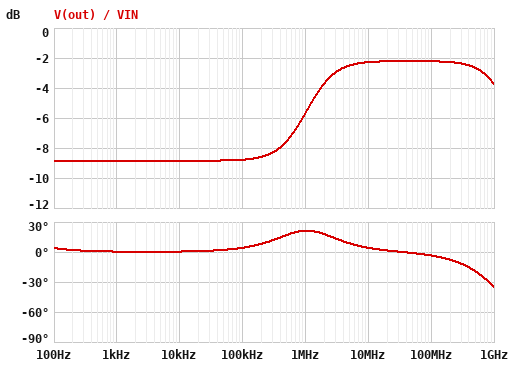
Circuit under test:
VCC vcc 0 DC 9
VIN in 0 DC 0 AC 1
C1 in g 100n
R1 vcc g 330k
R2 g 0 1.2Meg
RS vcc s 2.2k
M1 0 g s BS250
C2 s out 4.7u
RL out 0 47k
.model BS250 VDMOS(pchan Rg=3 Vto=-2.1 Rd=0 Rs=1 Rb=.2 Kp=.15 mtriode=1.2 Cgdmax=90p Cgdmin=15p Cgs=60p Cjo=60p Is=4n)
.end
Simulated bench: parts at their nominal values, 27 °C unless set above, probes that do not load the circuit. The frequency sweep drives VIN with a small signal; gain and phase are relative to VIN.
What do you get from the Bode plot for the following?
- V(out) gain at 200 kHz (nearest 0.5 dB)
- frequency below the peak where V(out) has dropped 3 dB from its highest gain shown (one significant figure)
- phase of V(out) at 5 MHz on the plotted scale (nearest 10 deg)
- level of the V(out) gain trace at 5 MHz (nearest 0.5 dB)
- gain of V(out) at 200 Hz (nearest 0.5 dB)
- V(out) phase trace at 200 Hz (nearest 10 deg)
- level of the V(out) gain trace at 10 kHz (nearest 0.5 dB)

-8.5 dB
1 MHz
10 deg
-2.5 dB
-9.0 dB
0 deg
-9.0 dB
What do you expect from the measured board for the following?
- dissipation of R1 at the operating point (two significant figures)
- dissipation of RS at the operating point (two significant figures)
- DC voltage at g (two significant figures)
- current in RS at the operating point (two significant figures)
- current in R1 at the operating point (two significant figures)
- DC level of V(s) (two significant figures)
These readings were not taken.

11 µW
460 nW
7.1 V
14 µA
5.9 µA
9.0 V
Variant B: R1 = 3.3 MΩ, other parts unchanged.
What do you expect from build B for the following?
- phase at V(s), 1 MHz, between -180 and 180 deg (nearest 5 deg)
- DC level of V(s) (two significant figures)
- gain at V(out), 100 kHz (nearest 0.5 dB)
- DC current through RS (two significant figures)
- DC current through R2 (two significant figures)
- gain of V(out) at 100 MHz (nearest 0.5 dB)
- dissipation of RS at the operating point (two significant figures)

0 deg
4.6 V
0 dB
2.0 mA
2.0 µA
-2.5 dB
8.6 mW
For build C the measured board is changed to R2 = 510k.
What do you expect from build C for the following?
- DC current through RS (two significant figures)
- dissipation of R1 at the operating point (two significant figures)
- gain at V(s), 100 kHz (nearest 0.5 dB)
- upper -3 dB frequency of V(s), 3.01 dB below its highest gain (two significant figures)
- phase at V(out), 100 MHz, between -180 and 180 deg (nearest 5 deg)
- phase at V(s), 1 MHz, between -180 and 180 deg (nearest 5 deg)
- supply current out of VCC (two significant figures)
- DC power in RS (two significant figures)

630 µA
38 µW
-0.5 dB
800 MHz
-5 deg
0 deg
640 µA
880 µW
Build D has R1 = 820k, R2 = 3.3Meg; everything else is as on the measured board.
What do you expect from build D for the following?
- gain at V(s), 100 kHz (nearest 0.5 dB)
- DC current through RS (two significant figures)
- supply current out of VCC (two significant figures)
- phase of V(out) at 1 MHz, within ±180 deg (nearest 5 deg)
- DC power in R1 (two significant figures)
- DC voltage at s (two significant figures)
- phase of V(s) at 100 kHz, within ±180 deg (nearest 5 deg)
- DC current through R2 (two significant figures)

-20.5 dB
1.4 µA
3.6 µA
40 deg
3.9 µW
9.0 V
50 deg
2.2 µA
